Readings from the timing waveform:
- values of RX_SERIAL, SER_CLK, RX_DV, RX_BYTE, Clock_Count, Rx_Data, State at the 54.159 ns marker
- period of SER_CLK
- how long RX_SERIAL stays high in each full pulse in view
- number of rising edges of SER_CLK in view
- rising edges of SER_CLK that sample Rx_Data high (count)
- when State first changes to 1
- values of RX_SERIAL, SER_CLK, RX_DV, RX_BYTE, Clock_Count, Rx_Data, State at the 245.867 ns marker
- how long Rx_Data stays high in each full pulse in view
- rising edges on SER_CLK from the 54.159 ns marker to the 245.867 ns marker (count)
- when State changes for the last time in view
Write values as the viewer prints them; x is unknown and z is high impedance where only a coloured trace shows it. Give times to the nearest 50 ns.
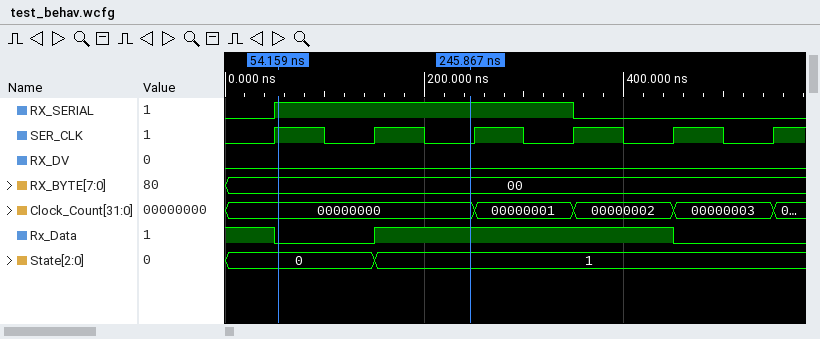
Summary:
RX_SERIAL=1, SER_CLK=1, RX_DV=0, RX_BYTE=00, Clock_Count=00000000, Rx_Data=0, State=0
100 ns
300 ns
6
4
150 ns
RX_SERIAL=1, SER_CLK=0, RX_DV=0, RX_BYTE=00, Clock_Count=00000000, Rx_Data=1, State=1
300 ns
1
150 ns
